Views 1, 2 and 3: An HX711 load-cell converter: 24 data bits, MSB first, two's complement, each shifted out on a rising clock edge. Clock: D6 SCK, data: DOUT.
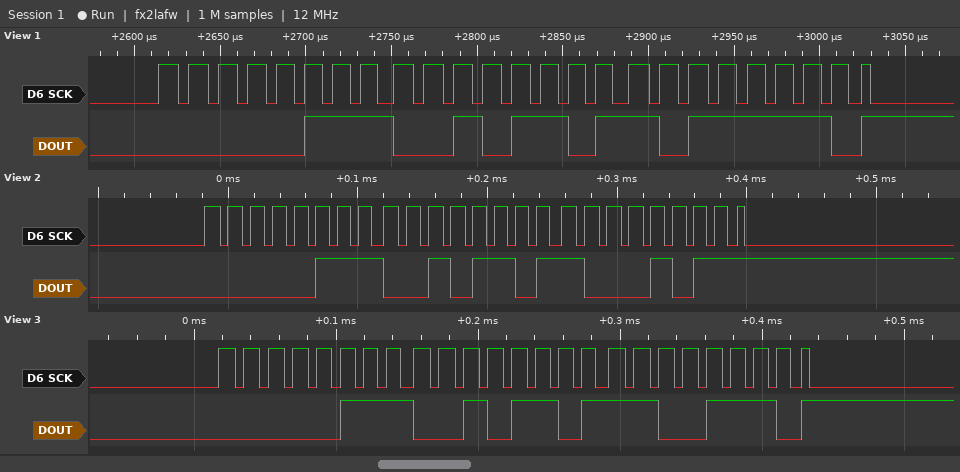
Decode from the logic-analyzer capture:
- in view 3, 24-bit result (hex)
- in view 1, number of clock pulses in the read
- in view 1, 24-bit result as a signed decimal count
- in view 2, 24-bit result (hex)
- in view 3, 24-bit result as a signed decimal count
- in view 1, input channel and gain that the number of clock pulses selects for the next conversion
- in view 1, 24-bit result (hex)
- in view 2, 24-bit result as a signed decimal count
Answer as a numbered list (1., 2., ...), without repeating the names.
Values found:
1. 0x072DCE
2. 25
3. 470462
4. 0x072D8B
5. 470478
6. channel A, gain 128
7. 0x072DBE
8. 470411
